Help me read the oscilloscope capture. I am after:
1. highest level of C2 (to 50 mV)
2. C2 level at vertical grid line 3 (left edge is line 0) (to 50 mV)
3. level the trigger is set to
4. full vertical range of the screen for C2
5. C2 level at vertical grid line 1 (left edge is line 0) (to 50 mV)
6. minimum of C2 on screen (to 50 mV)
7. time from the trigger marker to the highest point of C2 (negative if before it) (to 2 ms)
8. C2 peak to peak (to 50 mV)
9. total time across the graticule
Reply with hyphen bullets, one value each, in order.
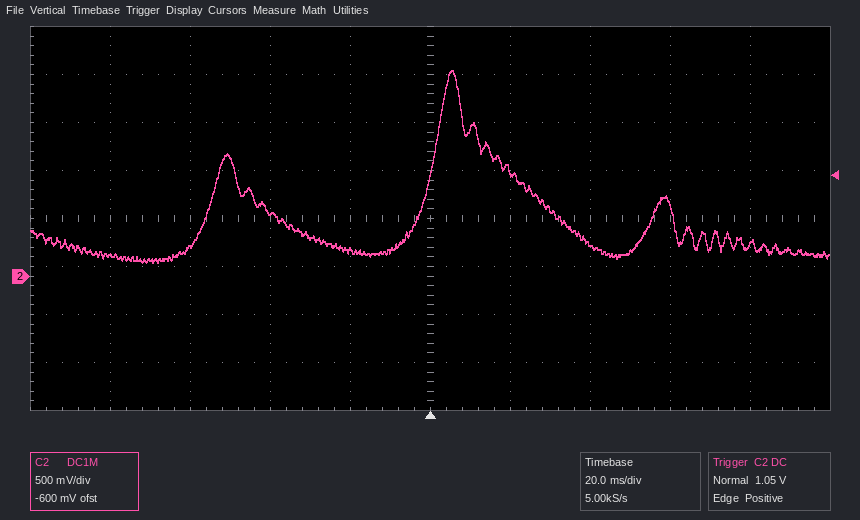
- 2.15 V
- 650 mV
- 1.05 V
- 4 V
- 200 mV
- 150 mV
- +6 ms
- 2.00 V
- 200 ms
